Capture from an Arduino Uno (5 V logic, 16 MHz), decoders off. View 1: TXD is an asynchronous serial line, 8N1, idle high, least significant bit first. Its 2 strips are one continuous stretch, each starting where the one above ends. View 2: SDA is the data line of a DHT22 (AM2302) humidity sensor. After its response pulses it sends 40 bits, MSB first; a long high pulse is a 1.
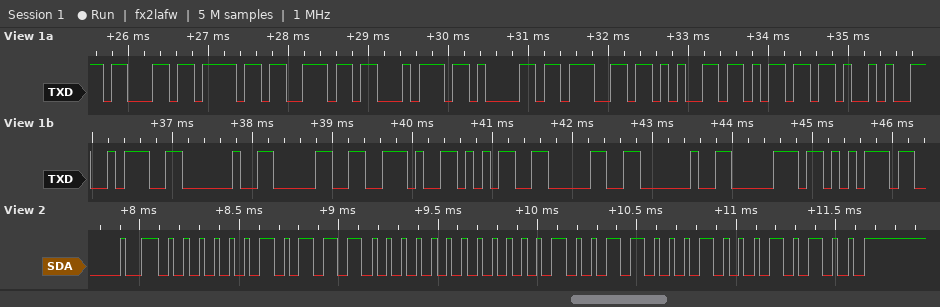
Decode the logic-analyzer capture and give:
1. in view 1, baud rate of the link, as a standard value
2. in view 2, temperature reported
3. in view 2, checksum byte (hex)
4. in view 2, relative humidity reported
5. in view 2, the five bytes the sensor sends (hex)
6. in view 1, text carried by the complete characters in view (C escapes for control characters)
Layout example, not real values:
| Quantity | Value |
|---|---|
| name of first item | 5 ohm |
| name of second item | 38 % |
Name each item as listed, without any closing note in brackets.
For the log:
| Quantity | Value |
|---|---|
| in view 1, baud rate of the link, as a standard value | 9600 baud |
| in view 2, temperature reported | 30.5 °C |
| in view 2, checksum byte | 0x14 |
| in view 2, relative humidity reported | 73.6 % |
| in view 2, the five bytes the sensor sends | 02 E0 01 31 14 |
| in view 1, text carried by the complete characters in view | "contagem): 0.50 pu" |
